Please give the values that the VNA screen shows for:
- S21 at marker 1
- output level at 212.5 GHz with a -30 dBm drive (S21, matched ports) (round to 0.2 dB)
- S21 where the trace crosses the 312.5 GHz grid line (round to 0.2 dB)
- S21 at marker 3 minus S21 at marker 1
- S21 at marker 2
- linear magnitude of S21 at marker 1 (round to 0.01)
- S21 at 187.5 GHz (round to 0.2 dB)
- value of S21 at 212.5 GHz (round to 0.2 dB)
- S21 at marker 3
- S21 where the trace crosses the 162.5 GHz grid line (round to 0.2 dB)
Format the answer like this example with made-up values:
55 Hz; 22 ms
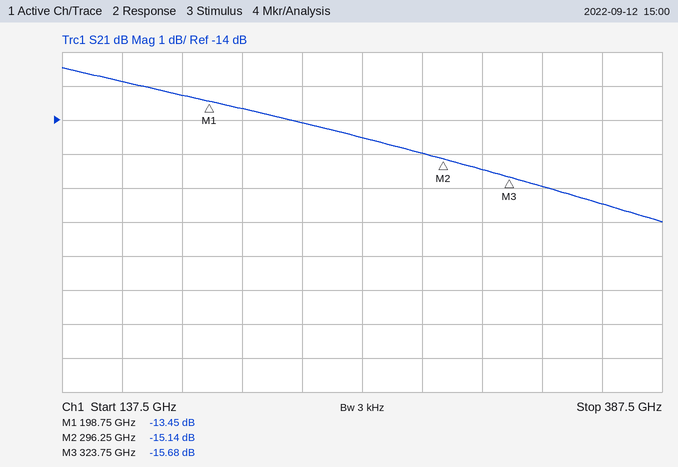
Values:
-13.45 dB; -43.6 dBm; -15.4 dB; -2.23 dB; -15.14 dB; 0.21; -13.2 dB; -13.6 dB; -15.68 dB; -12.8 dB
